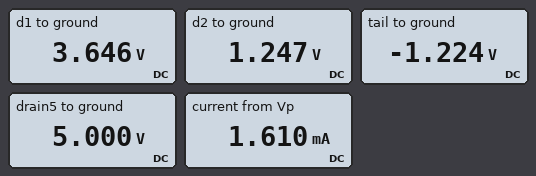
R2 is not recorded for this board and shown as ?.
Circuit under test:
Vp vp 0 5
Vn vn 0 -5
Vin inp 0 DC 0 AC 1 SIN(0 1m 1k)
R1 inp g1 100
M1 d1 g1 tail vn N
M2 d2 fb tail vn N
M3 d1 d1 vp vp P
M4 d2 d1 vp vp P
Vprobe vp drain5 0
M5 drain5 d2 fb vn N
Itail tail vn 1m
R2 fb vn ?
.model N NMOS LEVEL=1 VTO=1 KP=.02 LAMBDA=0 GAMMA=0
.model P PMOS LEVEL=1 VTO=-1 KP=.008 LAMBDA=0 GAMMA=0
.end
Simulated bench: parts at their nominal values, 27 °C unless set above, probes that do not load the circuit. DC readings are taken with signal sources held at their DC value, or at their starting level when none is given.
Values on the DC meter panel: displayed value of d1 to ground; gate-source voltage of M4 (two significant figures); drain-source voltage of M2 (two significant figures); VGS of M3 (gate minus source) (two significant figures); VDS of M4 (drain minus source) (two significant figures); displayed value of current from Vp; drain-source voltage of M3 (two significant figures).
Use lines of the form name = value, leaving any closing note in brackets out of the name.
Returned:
displayed value of d1 to ground = 3.646 V
gate-source voltage of M4 = -1.4 V
drain-source voltage of M2 = 2.5 V
VGS of M3 (gate minus source) = -1.4 V
VDS of M4 (drain minus source) = -3.8 V
displayed value of current from Vp = 1.610 mA
drain-source voltage of M3 = -1.4 V
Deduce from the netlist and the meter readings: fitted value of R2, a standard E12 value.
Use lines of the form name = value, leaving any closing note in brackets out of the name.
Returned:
fitted value of R2, a standard E12 value = 8.2 kΩ
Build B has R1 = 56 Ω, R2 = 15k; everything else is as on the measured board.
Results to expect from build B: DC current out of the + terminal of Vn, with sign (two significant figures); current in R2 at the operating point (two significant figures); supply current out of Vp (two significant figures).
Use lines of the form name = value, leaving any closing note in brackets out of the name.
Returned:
DC current out of the + terminal of Vn, with sign = -1.3 mA
current in R2 at the operating point = 330 µA
supply current out of Vp = 1.3 mA
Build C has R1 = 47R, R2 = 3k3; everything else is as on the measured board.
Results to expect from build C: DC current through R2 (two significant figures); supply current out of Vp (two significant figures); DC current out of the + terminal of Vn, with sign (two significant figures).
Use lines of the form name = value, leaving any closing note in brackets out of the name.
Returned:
DC current through R2 = 1.5 mA
supply current out of Vp = 2.5 mA
DC current out of the + terminal of Vn, with sign = -2.5 mA
